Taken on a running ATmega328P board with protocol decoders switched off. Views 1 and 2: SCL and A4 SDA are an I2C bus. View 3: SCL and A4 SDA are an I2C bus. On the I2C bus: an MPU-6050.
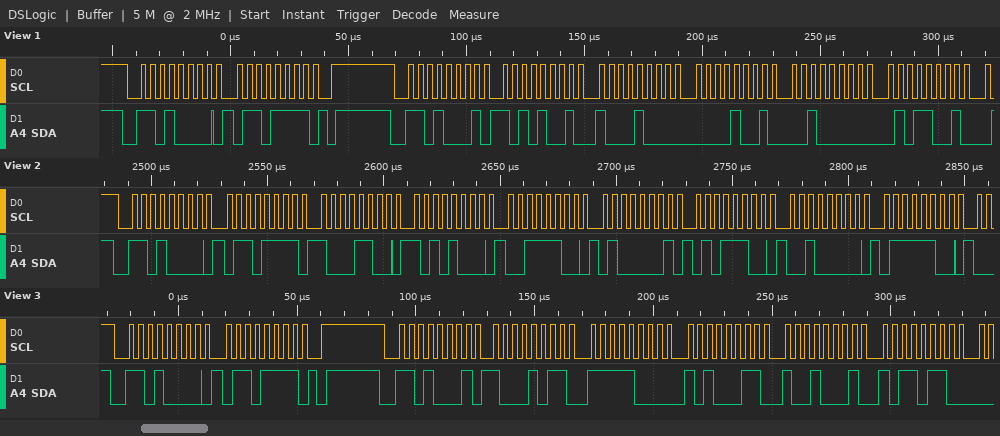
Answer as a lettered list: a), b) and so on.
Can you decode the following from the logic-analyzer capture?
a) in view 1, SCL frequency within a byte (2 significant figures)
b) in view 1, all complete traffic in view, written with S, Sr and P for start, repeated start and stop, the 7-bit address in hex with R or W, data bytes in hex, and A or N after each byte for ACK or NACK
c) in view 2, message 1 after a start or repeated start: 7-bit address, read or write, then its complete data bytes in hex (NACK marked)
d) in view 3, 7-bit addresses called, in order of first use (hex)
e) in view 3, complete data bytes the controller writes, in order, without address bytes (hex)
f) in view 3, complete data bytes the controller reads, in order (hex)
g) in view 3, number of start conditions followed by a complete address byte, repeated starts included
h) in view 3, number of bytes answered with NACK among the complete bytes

a) 250 kHz
b) S 68W A 6F A P S 68R A A9 A 88 A 09 A 20 A 59 A
c) 0x68 write: 6F 8C A8 3C 41 5C 20 7C
d) 0x68
e) 6F
f) 8B F8 A3 91 B6
g) 2
h) 0
